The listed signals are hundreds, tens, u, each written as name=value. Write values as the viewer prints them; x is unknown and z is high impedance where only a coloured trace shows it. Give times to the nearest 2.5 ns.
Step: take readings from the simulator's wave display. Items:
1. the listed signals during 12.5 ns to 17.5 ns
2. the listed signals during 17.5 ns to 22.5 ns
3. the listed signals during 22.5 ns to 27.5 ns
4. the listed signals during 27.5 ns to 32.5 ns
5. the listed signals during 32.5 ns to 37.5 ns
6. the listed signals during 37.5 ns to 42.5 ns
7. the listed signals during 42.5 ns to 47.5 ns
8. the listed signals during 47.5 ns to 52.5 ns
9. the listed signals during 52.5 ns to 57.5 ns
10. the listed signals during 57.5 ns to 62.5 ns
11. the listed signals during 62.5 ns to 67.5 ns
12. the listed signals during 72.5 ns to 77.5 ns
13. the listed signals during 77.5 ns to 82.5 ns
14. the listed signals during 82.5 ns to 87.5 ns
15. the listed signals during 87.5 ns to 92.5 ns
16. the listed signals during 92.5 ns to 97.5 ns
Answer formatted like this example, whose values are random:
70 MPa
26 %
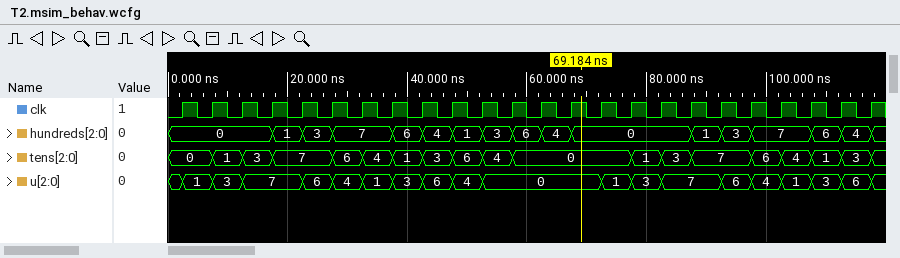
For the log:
hundreds=0, tens=3, u=7
hundreds=1, tens=7, u=7
hundreds=3, tens=7, u=6
hundreds=7, tens=6, u=4
hundreds=7, tens=4, u=1
hundreds=6, tens=1, u=3
hundreds=4, tens=3, u=6
hundreds=1, tens=6, u=4
hundreds=3, tens=4, u=0
hundreds=6, tens=0, u=0
hundreds=4, tens=0, u=0
hundreds=0, tens=0, u=1
hundreds=0, tens=1, u=3
hundreds=0, tens=3, u=7
hundreds=1, tens=7, u=7
hundreds=3, tens=7, u=6
